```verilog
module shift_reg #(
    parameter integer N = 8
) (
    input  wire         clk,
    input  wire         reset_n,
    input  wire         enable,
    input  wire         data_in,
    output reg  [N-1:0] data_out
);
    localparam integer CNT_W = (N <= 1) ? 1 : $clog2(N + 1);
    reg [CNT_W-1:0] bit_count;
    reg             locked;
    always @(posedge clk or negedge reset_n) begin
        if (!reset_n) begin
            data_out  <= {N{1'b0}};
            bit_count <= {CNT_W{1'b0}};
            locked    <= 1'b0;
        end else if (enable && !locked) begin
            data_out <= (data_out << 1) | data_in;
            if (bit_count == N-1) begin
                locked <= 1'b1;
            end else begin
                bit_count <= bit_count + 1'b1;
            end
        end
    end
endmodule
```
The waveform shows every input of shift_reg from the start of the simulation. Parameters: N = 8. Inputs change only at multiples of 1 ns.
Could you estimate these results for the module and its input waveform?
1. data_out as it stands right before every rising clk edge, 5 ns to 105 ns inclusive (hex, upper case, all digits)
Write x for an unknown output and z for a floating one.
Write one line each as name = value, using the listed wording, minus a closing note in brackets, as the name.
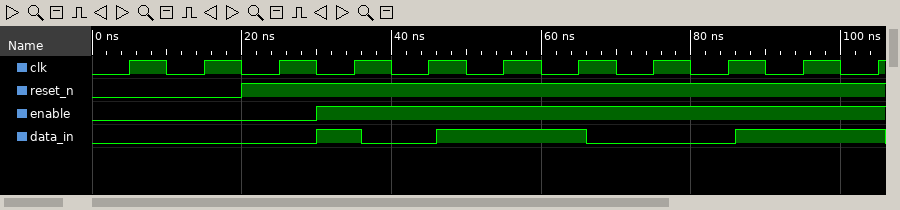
data_out as it stands right before every rising clk edge, 5 ns to 105 ns inclusive = 00, 00, 00, 00, 01, 02, 05, 0B, 16, 2C, 59
